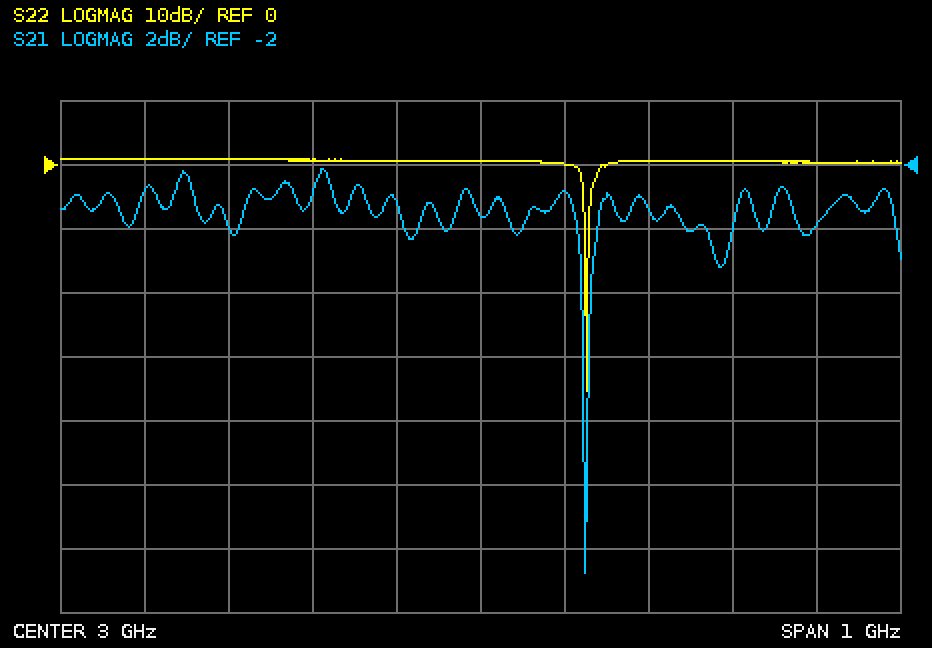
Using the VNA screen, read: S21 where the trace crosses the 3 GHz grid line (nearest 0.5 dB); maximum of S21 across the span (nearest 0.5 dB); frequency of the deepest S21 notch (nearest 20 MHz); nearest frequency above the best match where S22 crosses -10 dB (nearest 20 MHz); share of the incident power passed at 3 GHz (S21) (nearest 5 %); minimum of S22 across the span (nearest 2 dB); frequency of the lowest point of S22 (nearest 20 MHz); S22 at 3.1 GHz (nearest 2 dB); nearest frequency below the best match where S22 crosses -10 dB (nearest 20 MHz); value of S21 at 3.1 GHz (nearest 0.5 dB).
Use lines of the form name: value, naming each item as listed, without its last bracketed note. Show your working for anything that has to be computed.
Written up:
S21 where the trace crosses the 3 GHz grid line: -3.5 dB
maximum of S21 across the span: -2.0 dB
frequency of the deepest S21 notch: 3.12 GHz
nearest frequency above the best match where S22 crosses -10 dB: 3.12 GHz
share of the incident power passed at 3 GHz (S21): 10^(-3.5/10) ≈ 45 %
minimum of S22 across the span: -36 dB
frequency of the lowest point of S22: 3.12 GHz
S22 at 3.1 GHz: 0 dB
nearest frequency below the best match where S22 crosses -10 dB: 3.12 GHz
value of S21 at 3.1 GHz: -3.0 dB
